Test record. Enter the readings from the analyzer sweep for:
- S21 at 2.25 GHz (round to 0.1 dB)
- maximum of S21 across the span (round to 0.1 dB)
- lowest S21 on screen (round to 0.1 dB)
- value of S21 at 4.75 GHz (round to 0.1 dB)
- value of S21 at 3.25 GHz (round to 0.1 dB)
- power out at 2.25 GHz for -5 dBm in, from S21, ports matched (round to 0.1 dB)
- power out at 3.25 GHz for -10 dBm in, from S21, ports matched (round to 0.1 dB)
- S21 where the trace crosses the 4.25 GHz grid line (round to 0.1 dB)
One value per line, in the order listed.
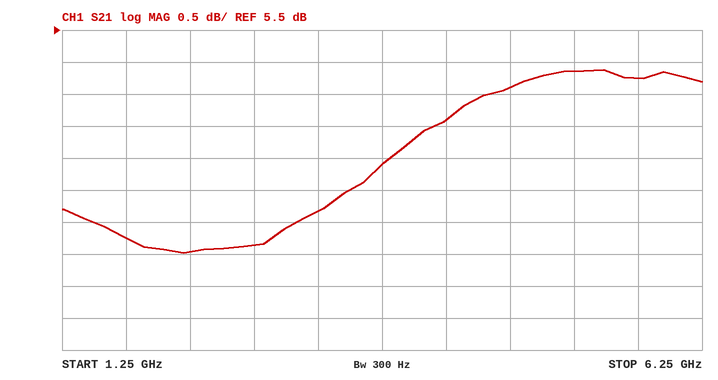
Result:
2.0 dB
4.9 dB
2.0 dB
4.6 dB
2.7 dB
-3.0 dBm
-7.3 dBm
4.1 dB
